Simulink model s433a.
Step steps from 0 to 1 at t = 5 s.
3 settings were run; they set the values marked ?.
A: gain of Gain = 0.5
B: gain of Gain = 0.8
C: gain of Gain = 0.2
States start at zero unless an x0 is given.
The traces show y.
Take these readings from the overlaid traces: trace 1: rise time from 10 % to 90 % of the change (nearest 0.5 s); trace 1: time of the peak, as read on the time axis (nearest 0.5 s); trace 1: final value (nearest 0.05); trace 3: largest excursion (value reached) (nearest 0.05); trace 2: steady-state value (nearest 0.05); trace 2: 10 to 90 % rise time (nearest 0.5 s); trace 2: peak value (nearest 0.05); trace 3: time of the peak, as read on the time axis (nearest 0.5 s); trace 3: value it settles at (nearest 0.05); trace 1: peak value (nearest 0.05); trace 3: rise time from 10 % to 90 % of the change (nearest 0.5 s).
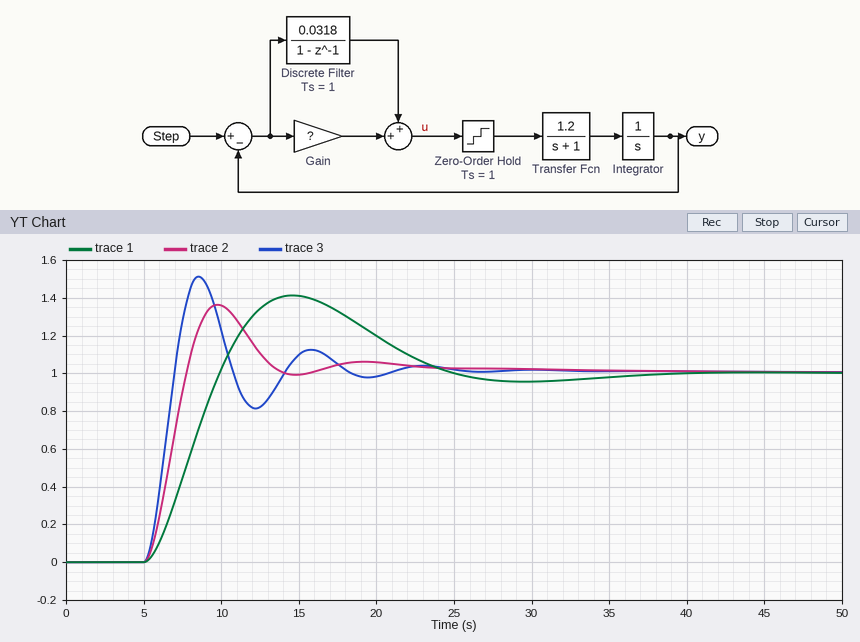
3.5 s
14.5 s
1.00
1.50
1.00
2.0 s
1.35
8.5 s
1.00
1.40
1.5 s
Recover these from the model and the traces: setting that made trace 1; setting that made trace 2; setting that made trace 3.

C
A
B
